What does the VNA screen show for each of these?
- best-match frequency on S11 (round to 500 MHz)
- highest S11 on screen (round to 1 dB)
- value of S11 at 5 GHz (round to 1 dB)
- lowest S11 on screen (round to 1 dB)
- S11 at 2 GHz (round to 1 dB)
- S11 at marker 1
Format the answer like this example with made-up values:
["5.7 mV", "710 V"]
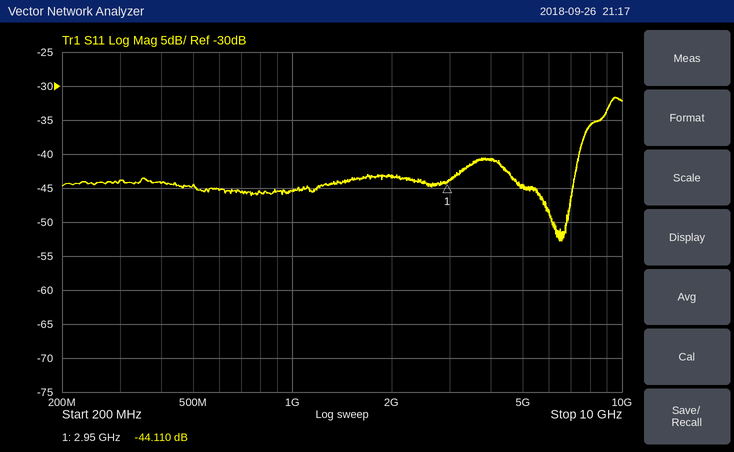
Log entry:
["6.5 GHz", "-32 dB", "-45 dB", "-53 dB", "-43 dB", "-44.110 dB"]
